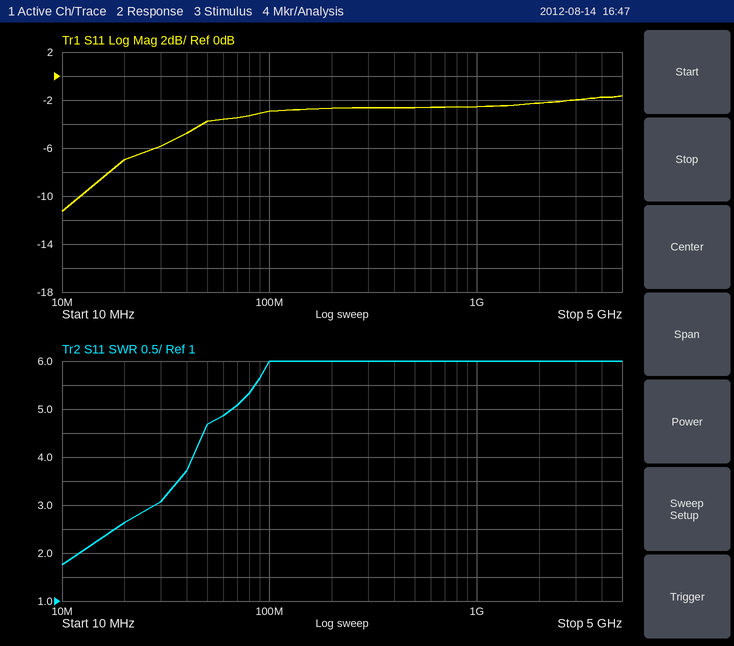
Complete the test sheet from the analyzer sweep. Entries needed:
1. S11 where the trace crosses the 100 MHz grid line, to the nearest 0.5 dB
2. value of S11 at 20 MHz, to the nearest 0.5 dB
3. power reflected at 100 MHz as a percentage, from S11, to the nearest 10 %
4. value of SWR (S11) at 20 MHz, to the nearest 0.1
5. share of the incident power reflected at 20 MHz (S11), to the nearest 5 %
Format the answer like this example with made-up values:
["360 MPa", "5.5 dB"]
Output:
["-3.0 dB", "-7.0 dB", "50 %", "2.6", "20 %"]
